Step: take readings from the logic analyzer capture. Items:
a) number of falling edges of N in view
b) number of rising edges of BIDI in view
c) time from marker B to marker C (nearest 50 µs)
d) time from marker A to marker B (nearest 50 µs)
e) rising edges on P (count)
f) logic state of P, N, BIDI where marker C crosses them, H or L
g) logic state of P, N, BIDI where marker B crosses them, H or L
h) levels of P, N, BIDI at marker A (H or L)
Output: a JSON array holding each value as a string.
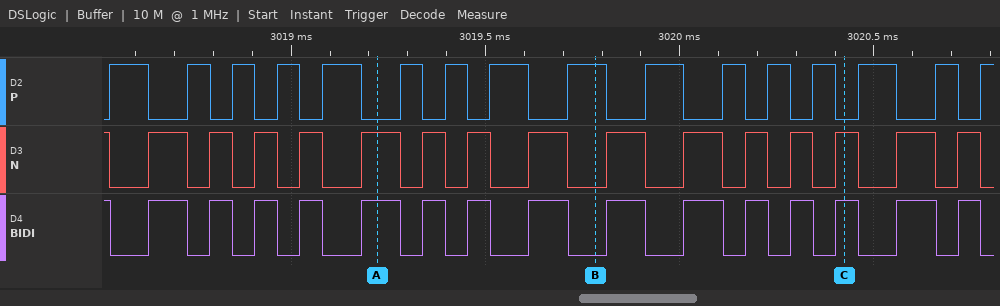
["16", "15", "650 µs", "550 µs", "16", "P=L, N=H, BIDI=H", "P=H, N=L, BIDI=L", "P=L, N=H, BIDI=H"]
